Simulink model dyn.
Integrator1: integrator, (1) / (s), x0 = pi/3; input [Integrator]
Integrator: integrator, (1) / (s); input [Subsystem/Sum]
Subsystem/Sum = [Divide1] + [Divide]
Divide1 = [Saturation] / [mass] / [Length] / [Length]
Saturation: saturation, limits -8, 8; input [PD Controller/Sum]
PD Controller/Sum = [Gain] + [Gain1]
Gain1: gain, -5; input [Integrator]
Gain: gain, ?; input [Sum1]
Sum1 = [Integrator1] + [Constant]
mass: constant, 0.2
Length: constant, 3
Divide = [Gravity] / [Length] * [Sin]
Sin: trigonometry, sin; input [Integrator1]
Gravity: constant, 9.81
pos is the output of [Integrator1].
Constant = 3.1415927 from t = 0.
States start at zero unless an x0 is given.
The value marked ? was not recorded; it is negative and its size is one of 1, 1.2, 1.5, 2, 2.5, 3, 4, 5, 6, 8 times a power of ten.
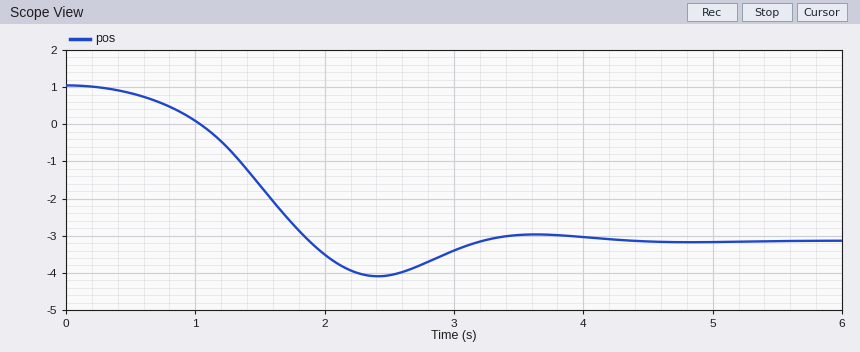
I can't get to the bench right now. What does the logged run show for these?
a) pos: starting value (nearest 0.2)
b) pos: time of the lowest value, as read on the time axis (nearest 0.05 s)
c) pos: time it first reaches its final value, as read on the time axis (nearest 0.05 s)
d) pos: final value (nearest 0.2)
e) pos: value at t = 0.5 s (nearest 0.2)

1.0
2.40 s
1.90 s
-3.2
0.8
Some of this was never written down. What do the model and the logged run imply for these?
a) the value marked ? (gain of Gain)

-10
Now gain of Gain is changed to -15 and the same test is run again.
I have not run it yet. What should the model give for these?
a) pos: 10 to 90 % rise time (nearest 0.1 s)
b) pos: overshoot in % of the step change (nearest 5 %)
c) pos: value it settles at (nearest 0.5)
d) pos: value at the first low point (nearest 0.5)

1.0 s
35 %
-3.0
-4.5
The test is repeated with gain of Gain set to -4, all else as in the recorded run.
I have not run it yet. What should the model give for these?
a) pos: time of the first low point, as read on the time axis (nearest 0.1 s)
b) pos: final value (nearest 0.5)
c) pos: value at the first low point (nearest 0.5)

3.1 s
-3.0
-3.5
